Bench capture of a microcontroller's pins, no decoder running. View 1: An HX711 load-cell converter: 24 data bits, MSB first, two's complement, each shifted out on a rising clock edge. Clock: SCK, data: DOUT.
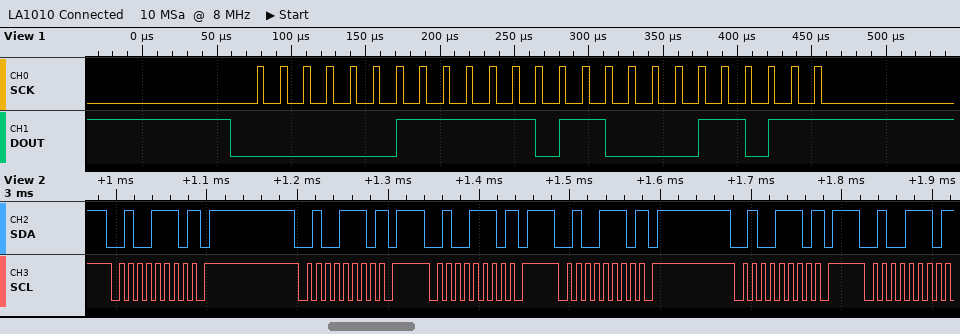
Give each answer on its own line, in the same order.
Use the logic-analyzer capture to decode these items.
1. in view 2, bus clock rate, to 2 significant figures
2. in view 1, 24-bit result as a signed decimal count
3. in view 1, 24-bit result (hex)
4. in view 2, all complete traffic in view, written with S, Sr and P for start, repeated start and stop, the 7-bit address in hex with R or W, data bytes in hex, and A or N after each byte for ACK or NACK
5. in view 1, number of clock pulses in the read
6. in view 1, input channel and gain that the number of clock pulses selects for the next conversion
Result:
100 kHz
259611
0x03F61B
S 27W N P S 27W N P S 27W N P S 27W N P S 27W N P S 27W N
25
channel A, gain 128
